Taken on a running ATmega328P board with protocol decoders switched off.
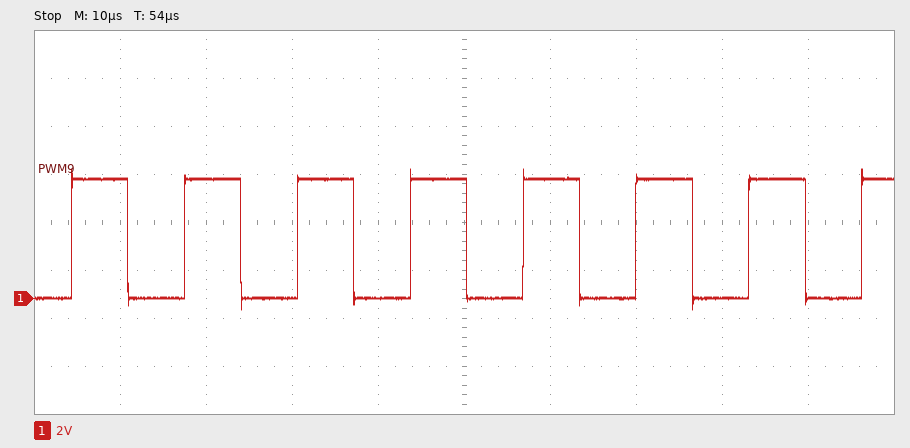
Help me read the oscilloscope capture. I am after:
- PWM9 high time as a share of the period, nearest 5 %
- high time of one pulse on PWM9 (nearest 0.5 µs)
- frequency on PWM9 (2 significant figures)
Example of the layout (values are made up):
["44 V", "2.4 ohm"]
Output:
["50 %", "6.5 µs", "76 kHz"]
